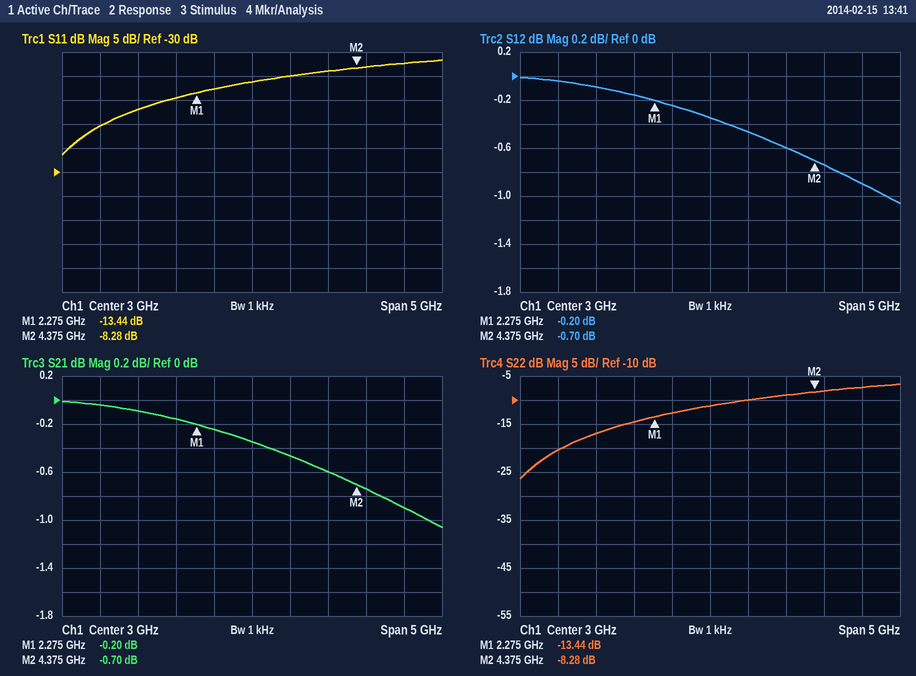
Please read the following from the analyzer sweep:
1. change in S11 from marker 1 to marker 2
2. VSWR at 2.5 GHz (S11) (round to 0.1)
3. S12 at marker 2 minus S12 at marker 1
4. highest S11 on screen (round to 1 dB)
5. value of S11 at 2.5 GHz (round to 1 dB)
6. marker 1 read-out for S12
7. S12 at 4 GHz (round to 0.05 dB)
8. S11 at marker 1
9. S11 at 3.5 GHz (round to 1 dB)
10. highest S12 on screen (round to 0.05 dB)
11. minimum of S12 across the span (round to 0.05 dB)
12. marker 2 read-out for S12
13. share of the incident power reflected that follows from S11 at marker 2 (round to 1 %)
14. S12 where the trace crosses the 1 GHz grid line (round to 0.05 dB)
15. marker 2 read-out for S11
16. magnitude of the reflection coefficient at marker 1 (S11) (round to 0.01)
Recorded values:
5.16 dB
1.6
-0.50 dB
-7 dB
-13 dB
-0.20 dB
-0.60 dB
-13.44 dB
-10 dB
0.00 dB
-1.05 dB
-0.70 dB
15 %
-0.05 dB
-8.28 dB
0.21
